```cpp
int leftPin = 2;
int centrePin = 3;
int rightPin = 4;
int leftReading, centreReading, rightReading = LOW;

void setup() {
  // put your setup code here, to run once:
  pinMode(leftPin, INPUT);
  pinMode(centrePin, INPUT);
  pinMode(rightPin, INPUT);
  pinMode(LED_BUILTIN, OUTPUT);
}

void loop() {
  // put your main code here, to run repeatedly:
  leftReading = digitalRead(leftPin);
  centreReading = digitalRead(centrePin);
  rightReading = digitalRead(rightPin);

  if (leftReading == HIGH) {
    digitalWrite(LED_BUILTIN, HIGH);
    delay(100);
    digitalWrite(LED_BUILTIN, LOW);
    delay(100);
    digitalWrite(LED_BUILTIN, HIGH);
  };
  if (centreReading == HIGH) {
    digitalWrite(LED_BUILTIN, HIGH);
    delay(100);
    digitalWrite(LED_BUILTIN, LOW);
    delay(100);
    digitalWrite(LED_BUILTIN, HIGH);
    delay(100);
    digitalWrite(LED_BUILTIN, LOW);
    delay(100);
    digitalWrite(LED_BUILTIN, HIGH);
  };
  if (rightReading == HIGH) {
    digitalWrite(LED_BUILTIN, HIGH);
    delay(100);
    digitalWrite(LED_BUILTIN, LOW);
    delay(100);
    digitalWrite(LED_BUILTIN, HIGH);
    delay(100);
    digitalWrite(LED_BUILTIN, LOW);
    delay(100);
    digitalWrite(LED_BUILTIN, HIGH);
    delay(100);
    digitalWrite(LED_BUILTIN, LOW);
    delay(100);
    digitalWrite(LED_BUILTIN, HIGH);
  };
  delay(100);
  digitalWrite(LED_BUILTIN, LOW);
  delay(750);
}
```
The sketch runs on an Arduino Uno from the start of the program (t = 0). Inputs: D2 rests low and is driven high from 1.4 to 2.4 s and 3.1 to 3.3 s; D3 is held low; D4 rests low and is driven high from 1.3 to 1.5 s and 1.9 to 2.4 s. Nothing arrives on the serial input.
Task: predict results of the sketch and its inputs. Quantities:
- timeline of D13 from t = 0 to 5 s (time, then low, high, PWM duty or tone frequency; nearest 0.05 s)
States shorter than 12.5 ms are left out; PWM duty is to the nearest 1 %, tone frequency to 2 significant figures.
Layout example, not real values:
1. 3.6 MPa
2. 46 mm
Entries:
1. 0 s low; 1.7 s high; 1.8 s low; 1.9 s high; 2 s low
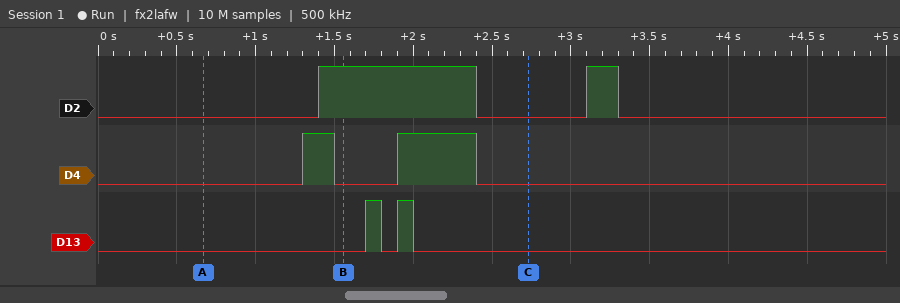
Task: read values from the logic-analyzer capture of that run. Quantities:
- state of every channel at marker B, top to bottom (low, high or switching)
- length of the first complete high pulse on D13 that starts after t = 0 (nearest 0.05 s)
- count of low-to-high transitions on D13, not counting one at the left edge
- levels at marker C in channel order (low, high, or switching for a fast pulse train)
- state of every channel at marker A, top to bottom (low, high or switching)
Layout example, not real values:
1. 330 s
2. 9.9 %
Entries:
1. D2 high, D4 low, D13 low
2. 0.10 s
3. 2
4. D2 low, D4 low, D13 low
5. D2 low, D4 low, D13 low
